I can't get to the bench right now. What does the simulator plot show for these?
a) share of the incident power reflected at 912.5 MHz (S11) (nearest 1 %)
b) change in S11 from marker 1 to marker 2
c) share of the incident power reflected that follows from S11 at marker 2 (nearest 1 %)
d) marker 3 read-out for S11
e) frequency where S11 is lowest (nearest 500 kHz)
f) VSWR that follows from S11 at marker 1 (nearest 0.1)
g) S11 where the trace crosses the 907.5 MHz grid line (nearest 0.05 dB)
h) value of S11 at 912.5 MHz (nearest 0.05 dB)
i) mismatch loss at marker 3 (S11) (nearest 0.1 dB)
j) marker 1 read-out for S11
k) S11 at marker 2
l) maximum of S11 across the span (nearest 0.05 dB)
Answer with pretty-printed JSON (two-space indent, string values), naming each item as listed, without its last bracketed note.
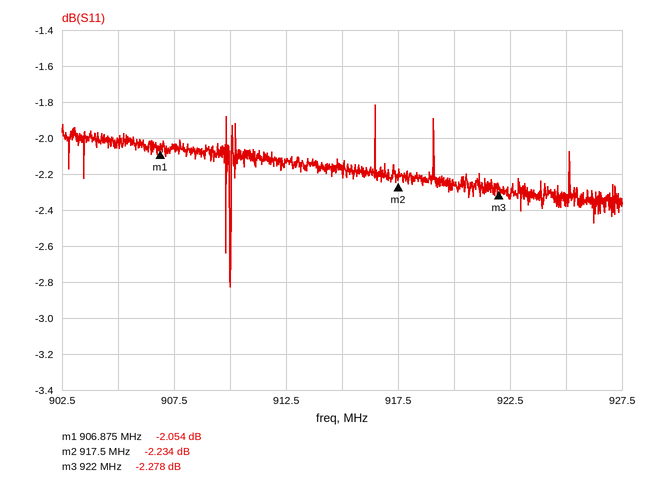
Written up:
{
  "share of the incident power reflected at 912.5 MHz (S11)": "61 %",
  "change in S11 from marker 1 to marker 2": "-0.180 dB",
  "share of the incident power reflected that follows from S11 at marker 2": "60 %",
  "marker 3 read-out for S11": "-2.278 dB",
  "frequency where S11 is lowest": "910.0 MHz",
  "VSWR that follows from S11 at marker 1": "8.5",
  "S11 where the trace crosses the 907.5 MHz grid line": "-2.05 dB",
  "value of S11 at 912.5 MHz": "-2.15 dB",
  "mismatch loss at marker 3 (S11)": "3.9 dB",
  "marker 1 read-out for S11": "-2.054 dB",
  "S11 at marker 2": "-2.234 dB",
  "maximum of S11 across the span": "-1.80 dB"
}
